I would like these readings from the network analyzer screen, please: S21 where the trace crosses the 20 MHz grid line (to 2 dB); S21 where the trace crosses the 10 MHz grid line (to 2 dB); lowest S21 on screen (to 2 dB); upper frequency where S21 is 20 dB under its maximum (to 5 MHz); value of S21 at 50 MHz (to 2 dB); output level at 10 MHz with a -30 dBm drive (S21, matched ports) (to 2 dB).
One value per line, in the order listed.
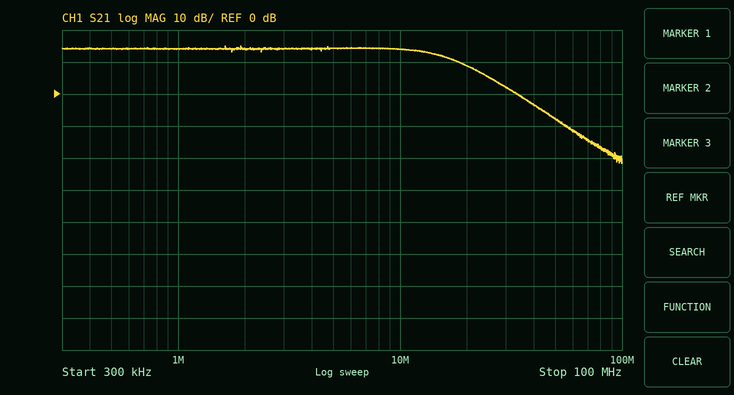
8 dB
14 dB
-22 dB
45 MHz
-8 dB
-16 dBm
